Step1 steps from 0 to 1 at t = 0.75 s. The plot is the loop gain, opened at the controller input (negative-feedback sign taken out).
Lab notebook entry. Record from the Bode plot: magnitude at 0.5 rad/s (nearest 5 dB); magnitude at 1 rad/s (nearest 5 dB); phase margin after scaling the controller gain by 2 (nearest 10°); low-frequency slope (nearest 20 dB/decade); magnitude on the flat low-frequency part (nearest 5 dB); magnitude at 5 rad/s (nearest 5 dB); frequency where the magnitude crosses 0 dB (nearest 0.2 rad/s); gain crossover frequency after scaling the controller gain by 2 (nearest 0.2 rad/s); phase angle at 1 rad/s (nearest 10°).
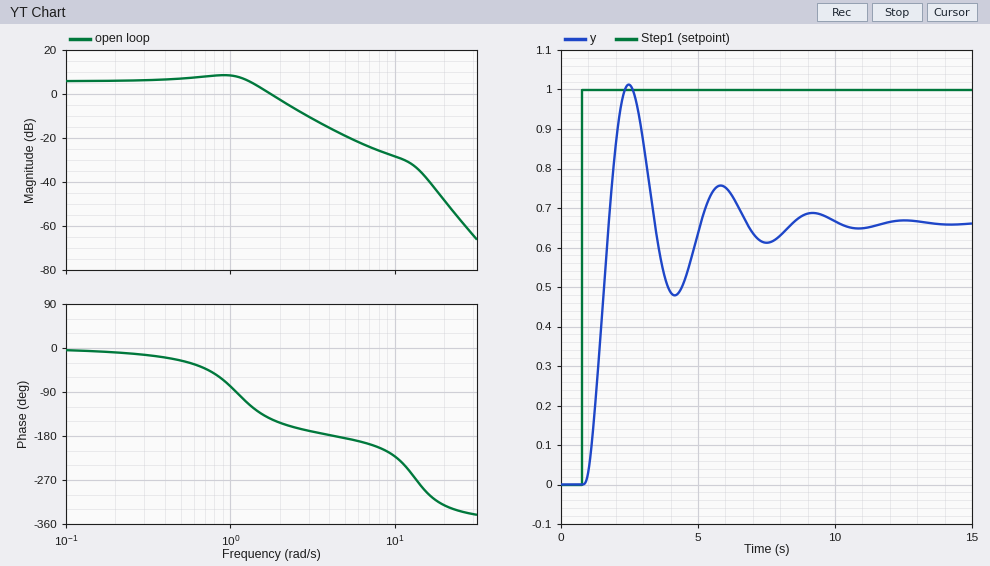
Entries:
5 dB
10 dB
20°
0 dB/decade
5 dB
-20 dB
1.8 rad/s
2.4 rad/s
-80°
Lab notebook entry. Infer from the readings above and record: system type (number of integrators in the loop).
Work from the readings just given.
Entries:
0
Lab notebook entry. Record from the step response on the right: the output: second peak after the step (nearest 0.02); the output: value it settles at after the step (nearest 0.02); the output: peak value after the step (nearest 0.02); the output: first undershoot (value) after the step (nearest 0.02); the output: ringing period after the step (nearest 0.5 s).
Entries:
0.76
0.66
1.02
0.48
3.5 s
